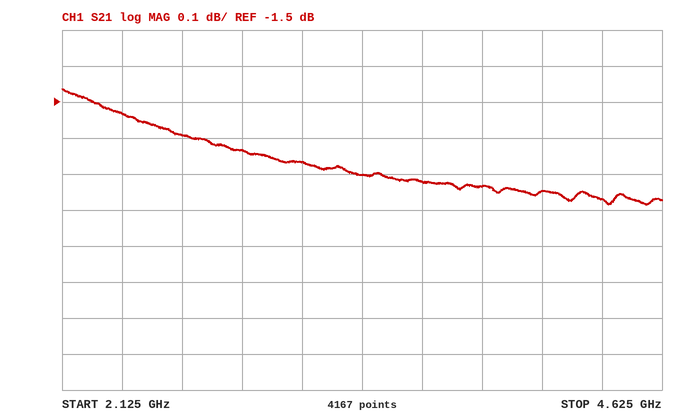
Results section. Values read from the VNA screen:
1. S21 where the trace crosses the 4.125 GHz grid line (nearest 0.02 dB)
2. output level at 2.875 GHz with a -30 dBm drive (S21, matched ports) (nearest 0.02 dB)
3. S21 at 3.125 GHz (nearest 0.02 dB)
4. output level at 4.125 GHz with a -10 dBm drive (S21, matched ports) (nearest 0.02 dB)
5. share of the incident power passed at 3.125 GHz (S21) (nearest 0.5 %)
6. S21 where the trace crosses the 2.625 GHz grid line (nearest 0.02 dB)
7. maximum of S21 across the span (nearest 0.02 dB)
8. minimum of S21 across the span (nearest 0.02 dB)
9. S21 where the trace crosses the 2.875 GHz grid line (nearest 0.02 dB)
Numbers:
-1.74 dB
-31.64 dBm
-1.66 dB
-11.74 dBm
68.0 %
-1.60 dB
-1.46 dB
-1.78 dB
-1.64 dB
